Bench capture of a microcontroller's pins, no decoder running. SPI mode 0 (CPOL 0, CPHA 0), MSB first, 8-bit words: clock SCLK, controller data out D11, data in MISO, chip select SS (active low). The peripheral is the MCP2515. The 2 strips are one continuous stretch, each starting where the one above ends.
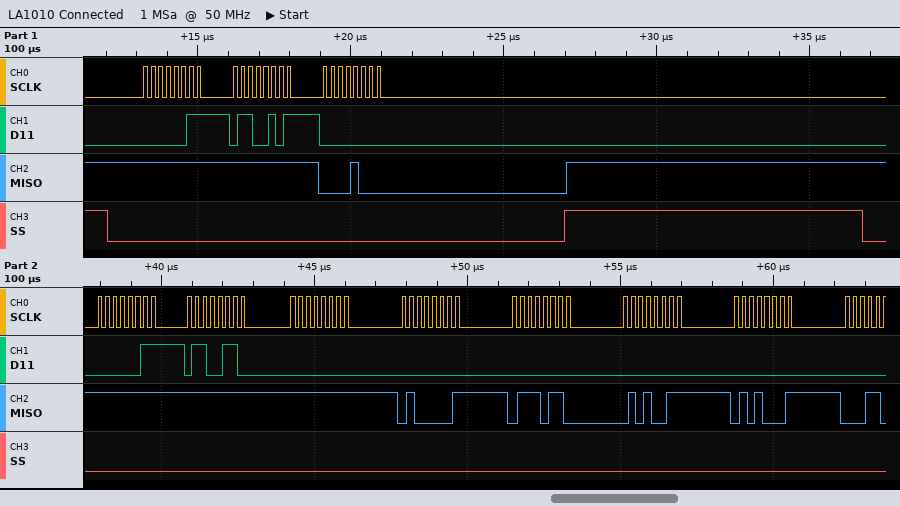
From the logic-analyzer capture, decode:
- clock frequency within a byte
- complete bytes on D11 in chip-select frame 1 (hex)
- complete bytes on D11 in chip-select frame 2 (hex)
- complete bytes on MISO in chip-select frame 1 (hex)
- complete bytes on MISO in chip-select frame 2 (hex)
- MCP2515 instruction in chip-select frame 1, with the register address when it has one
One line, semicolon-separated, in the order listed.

4 MHz; 03 65 00; 03 66 00 00 00 00 00; FF FF 08; FF FF FF 41 76 53 51; READ 0x65
